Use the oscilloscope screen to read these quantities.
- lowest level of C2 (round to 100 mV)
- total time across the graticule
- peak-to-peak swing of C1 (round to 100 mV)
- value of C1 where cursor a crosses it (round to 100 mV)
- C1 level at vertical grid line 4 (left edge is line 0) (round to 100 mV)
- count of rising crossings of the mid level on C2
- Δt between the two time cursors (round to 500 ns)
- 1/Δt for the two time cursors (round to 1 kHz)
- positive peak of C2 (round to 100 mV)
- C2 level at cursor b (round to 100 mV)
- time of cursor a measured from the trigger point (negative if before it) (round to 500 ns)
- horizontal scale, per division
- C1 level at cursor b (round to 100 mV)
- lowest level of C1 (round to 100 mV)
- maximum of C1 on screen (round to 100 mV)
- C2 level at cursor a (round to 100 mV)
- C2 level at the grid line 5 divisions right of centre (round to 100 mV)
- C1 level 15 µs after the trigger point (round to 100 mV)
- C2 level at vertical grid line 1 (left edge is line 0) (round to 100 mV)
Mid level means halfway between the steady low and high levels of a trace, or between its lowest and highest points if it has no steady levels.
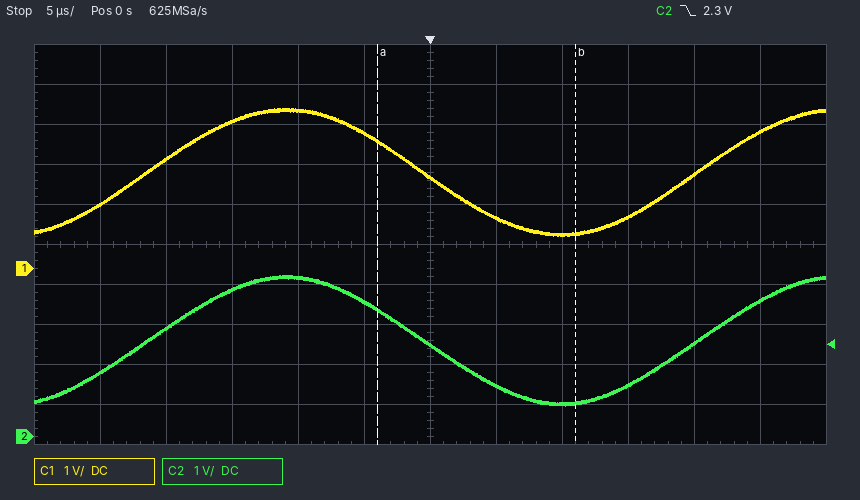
800 mV
60 µs
3.2 V
3.2 V
4.0 V
2
15.0 µs
67 kHz
4.0 V
800 mV
-4.0 µs
5 µs
900 mV
800 mV
4.0 V
3.2 V
3.4 V
1.3 V
1.6 V
